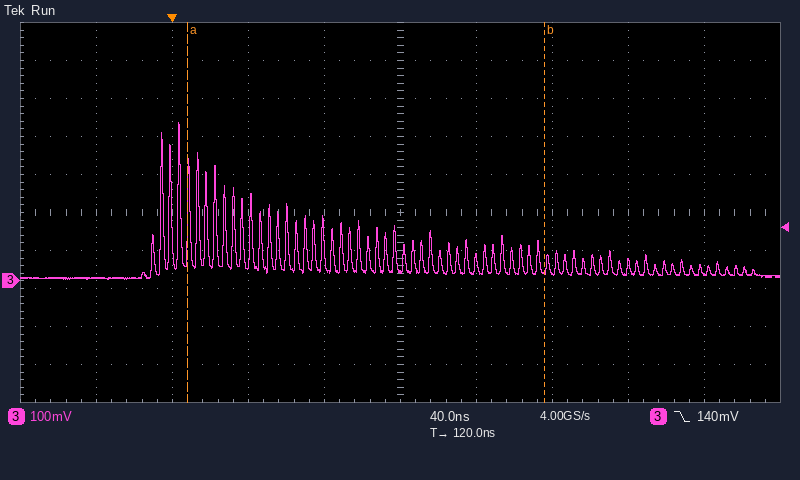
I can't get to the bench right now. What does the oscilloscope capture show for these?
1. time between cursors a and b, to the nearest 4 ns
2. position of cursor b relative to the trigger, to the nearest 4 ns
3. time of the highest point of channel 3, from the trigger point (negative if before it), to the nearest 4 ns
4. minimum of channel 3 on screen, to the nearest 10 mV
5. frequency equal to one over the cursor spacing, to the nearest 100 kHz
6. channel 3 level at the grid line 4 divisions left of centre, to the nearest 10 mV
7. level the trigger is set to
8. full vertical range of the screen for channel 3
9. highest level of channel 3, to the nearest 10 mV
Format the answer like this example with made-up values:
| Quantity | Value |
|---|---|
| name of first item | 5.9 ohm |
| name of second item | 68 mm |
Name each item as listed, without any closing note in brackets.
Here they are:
| Quantity | Value |
|---|---|
| time between cursors a and b, to the nearest 4 ns | 188 ns |
| position of cursor b relative to the trigger, to the nearest 4 ns | +196 ns |
| time of the highest point of channel 3, from the trigger point (negative if before it), to the nearest 4 ns | +4 ns |
| minimum of channel 3 on screen, to the nearest 10 mV | 0 mV |
| frequency equal to one over the cursor spacing, to the nearest 100 kHz | 5.3 MHz |
| channel 3 level at the grid line 4 divisions left of centre, to the nearest 10 mV | 10 mV |
| level the trigger is set to | 140 mV |
| full vertical range of the screen for channel 3 | 1 V |
| highest level of channel 3, to the nearest 10 mV | 420 mV |
